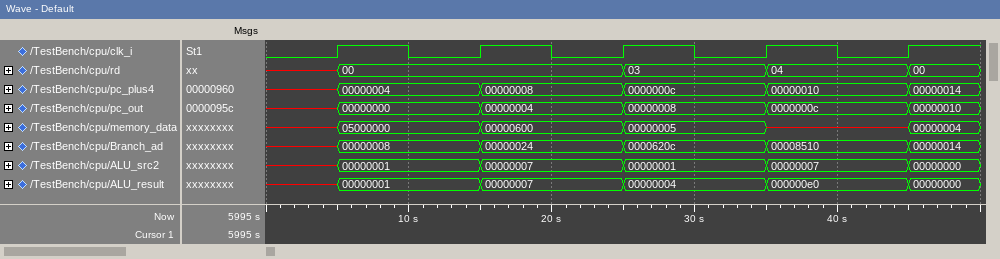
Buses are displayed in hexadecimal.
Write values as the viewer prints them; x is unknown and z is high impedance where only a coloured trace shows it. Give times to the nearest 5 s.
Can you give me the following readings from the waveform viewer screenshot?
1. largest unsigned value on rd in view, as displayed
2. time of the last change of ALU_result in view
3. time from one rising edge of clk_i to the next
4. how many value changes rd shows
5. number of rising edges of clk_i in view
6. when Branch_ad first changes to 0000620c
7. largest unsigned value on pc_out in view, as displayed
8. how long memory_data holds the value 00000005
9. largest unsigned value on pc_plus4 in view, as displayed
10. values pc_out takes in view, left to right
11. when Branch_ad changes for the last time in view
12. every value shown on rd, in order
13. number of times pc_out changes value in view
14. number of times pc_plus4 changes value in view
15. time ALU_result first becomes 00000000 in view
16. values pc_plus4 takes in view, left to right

04
45 s
10 s
4
5
25 s
00000010
10 s
00000014
x, 00000000, 00000004, 00000008, 0000000c, 00000010
45 s
x, 00, 03, 04, 00
5
5
45 s
x, 00000004, 00000008, 0000000c, 00000010, 00000014
